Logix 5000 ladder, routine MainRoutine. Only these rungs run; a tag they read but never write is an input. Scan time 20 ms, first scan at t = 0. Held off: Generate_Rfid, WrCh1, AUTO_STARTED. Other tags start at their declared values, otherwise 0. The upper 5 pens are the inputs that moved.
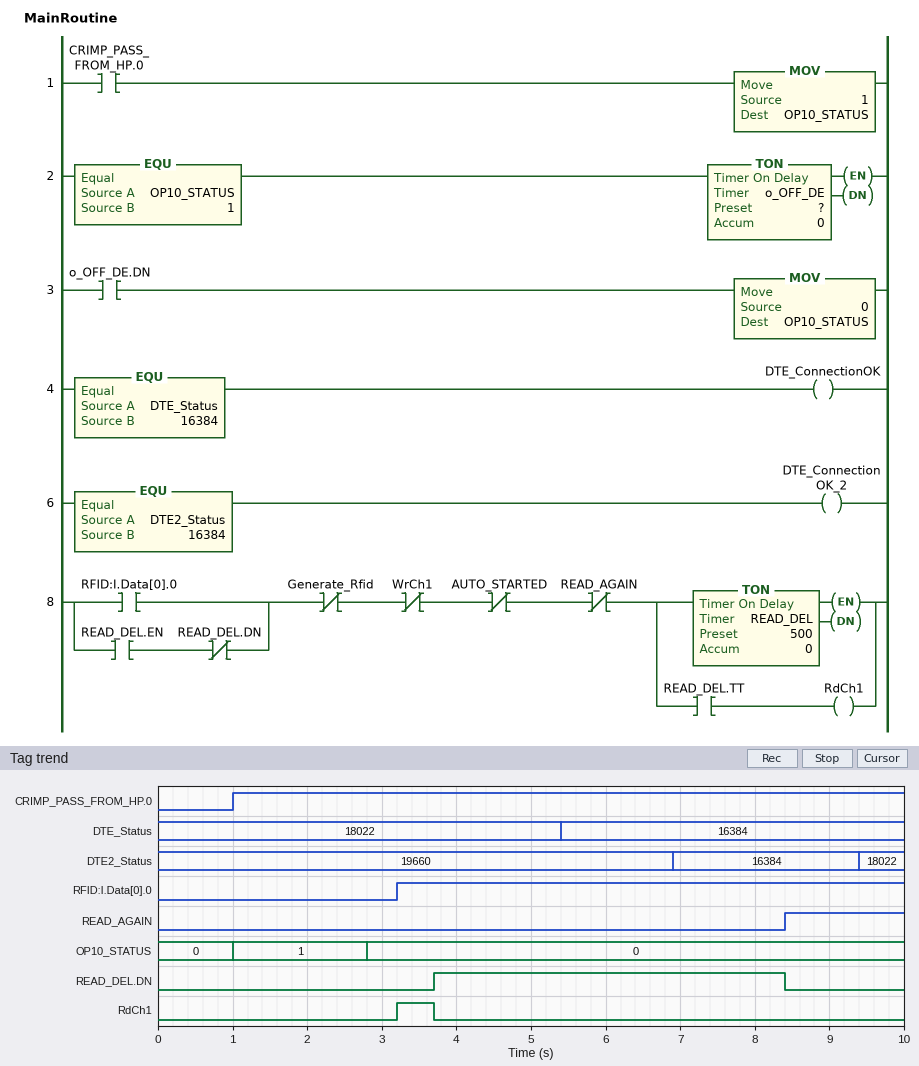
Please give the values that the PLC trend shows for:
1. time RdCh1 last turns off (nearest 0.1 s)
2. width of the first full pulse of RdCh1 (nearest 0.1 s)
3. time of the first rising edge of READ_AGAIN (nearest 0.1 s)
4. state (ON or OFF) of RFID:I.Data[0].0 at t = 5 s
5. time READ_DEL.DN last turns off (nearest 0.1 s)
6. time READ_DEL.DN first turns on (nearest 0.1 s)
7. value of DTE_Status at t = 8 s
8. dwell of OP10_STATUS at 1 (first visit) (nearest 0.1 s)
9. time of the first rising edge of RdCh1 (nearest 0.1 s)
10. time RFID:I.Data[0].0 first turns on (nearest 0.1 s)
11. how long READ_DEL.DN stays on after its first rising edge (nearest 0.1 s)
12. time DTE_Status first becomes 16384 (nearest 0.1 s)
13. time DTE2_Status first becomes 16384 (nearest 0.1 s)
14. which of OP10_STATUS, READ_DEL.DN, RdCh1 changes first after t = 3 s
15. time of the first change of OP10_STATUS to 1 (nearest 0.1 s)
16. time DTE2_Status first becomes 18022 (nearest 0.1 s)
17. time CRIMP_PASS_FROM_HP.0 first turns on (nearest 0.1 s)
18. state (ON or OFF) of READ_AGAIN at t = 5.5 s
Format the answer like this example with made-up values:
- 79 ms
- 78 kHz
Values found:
- 3.7 s
- 0.5 s
- 8.4 s
- ON
- 8.4 s
- 3.7 s
- 16384
- 1.8 s
- 3.2 s
- 3.2 s
- 4.7 s
- 5.4 s
- 6.9 s
- RdCh1
- 1.0 s
- 9.4 s
- 1.0 s
- OFF
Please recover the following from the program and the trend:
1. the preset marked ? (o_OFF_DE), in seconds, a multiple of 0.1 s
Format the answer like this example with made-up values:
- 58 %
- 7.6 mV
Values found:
- 1.8 s
